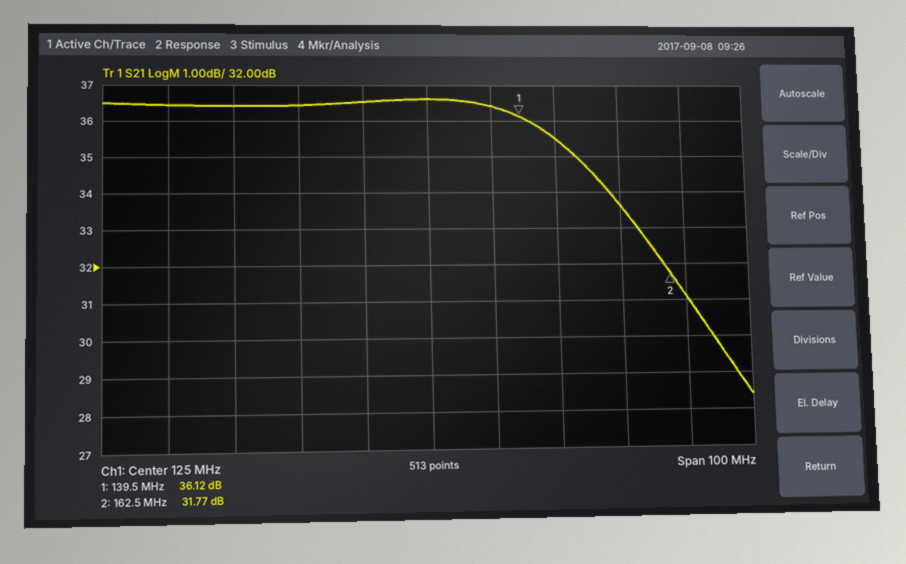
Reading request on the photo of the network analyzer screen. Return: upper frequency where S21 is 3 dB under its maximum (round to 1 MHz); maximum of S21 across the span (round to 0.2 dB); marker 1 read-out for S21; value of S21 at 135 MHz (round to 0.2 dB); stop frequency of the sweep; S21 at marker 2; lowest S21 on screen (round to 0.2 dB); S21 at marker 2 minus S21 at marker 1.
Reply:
155 MHz
36.6 dB
36.12 dB
36.4 dB
175 MHz
31.77 dB
28.4 dB
-4.35 dB
